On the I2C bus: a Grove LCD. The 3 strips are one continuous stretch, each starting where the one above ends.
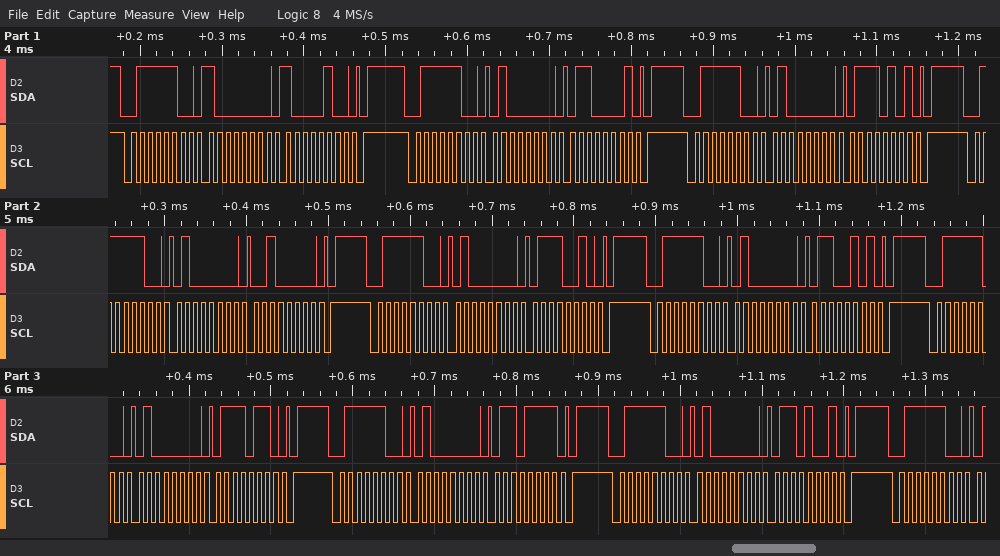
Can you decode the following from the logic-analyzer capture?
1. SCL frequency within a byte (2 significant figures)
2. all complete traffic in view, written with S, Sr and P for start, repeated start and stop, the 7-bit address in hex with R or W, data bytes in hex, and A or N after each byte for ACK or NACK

100 kHz
S 3EW A 80 A 84 A P S 3EW A 40 A 61 A P S 3EW A 40 A 75 A P S 3EW A 40 A 20 A P S 3EW A 40 A 72 A P S 3EW A 40 A 65 A P S 3EW A 40 A 76 A P S 3EW A 40 A 6F A P S 3EW A 40 A 69 A P S 3EW A
